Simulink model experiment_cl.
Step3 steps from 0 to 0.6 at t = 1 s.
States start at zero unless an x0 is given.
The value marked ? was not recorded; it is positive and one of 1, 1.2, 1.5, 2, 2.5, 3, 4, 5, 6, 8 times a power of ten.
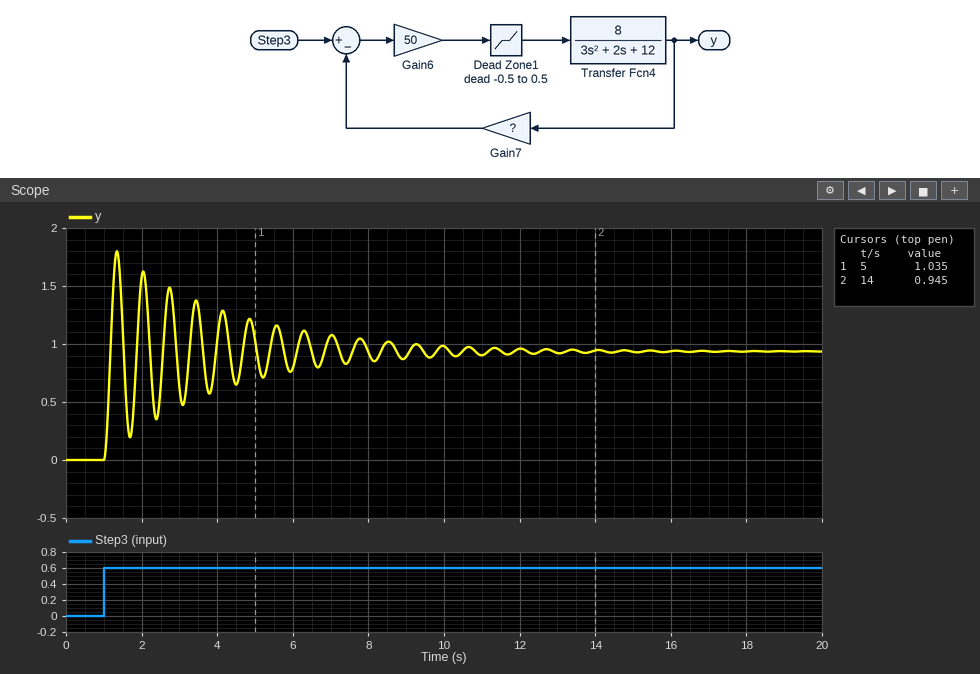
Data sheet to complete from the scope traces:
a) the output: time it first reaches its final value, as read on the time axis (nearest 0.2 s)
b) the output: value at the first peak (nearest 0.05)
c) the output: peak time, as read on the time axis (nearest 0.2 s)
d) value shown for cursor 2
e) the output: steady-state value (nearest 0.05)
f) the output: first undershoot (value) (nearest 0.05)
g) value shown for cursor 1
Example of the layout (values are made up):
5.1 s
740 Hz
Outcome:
1.2 s
1.80
1.4 s
0.945
0.95
0.20
1.035
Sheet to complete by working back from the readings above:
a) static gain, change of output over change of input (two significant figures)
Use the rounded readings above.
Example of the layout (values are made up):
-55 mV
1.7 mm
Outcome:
1.6
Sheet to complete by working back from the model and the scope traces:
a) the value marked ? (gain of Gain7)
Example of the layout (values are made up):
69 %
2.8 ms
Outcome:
0.6
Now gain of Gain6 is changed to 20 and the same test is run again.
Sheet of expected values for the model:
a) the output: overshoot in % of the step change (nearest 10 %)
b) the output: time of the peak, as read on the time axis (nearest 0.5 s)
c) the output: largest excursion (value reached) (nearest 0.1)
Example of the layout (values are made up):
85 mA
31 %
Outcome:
90 %
1.5 s
1.6
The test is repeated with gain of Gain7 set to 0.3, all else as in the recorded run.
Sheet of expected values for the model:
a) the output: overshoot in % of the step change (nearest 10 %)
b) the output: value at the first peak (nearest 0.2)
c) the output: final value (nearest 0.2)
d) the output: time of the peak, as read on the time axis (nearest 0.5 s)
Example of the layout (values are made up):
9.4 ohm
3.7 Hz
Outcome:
90 %
3.4
1.8
1.5 s
